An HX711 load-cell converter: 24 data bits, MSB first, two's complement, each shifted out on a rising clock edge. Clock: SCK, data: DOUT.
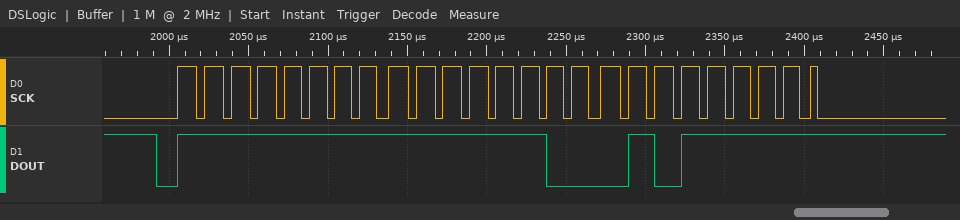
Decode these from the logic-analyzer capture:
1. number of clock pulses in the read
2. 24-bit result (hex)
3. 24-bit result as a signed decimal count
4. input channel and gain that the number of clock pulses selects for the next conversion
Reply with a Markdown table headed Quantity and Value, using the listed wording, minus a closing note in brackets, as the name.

| Quantity | Value |
|---|---|
| number of clock pulses in the read | 25 |
| 24-bit result | 0xFFFC5F |
| 24-bit result as a signed decimal count | -929 |
| input channel and gain that the number of clock pulses selects for the next conversion | channel A, gain 128 |
